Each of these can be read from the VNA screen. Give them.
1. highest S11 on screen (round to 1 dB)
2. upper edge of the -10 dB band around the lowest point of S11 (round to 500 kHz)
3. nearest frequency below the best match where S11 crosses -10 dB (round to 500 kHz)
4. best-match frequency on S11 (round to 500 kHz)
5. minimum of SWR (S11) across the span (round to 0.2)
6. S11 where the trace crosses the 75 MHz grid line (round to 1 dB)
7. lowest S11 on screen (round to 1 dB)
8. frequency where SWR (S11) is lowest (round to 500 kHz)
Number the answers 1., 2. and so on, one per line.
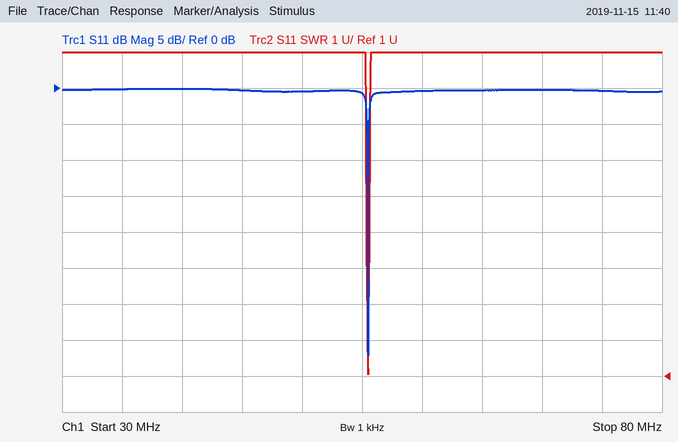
1. 0 dB
2. 55.5 MHz
3. 55.5 MHz
4. 55.5 MHz
5. 1.0
6. 0 dB
7. -37 dB
8. 55.5 MHz
